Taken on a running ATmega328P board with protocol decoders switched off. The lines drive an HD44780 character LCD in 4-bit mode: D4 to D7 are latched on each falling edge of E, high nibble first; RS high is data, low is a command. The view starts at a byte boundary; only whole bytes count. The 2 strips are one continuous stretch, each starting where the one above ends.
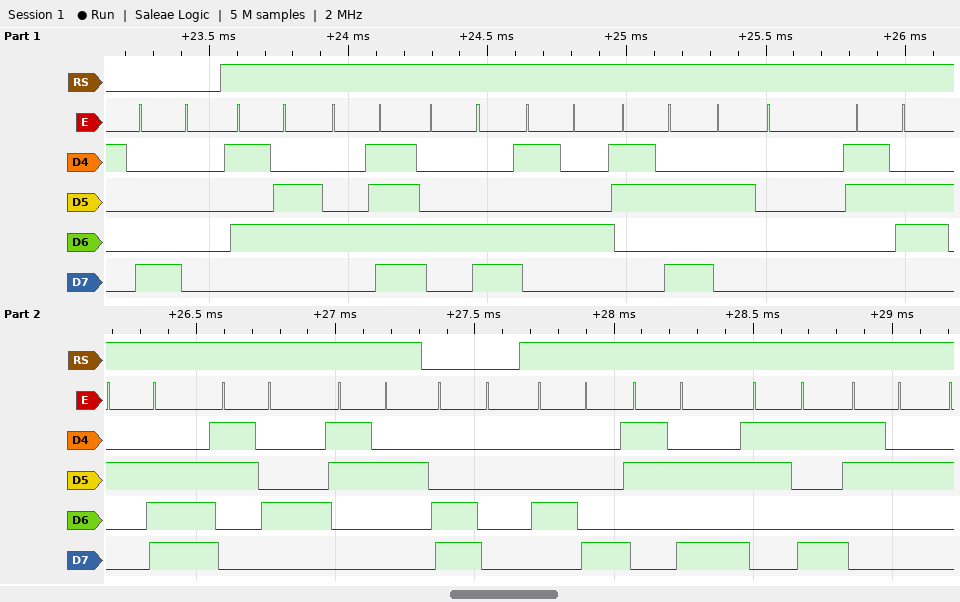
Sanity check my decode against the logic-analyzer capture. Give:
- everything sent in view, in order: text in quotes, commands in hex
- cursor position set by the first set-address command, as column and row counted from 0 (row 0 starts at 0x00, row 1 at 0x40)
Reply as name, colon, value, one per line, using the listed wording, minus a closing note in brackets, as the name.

everything sent in view, in order: text in quotes, commands in hex: 0x80 "VOLT: 6.42" 0xC0 "H:92"
cursor position set by the first set-address command, as column and row counted from 0: column 0, row 0
